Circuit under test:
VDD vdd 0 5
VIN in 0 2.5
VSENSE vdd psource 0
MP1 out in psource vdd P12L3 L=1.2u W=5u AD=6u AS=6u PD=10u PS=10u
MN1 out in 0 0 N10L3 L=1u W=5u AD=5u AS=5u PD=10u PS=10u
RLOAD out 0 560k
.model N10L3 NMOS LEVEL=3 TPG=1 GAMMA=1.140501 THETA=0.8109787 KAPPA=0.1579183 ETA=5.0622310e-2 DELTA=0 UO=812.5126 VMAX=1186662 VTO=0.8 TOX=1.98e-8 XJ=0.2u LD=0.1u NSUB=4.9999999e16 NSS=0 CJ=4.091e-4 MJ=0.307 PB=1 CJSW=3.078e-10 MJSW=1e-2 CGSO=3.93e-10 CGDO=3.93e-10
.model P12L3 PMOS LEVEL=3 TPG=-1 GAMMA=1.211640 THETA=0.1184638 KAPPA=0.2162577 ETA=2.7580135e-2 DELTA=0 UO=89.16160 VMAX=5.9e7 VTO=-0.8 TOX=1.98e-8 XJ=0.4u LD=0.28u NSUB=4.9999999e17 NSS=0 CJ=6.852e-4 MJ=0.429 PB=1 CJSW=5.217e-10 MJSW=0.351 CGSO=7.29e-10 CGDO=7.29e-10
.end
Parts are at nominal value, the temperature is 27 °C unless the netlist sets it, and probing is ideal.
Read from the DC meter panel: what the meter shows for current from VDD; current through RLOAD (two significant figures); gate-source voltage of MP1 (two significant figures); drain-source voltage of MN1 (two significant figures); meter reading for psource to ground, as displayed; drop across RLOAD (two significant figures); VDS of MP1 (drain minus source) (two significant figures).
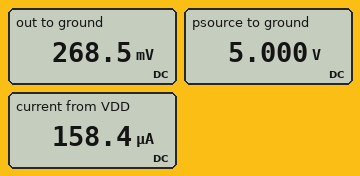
158.4 µA
480 nA
-2.5 V
270 mV
5.000 V
270 mV
-4.7 V
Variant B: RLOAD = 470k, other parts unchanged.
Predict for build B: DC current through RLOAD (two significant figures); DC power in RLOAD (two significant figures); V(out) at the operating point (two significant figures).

570 nA
150 nW
270 mV
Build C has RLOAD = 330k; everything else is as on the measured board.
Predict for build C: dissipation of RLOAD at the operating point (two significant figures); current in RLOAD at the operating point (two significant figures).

220 nW
810 nA
